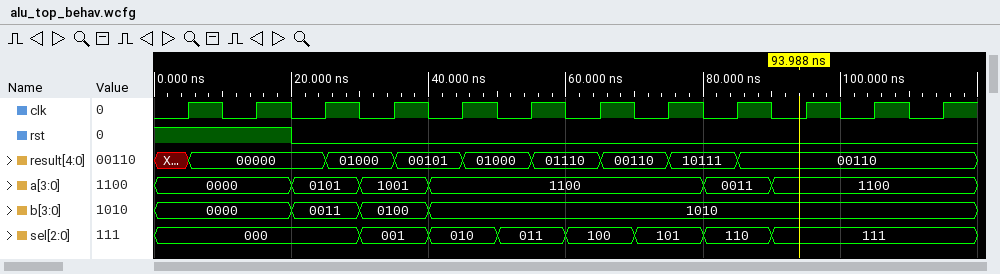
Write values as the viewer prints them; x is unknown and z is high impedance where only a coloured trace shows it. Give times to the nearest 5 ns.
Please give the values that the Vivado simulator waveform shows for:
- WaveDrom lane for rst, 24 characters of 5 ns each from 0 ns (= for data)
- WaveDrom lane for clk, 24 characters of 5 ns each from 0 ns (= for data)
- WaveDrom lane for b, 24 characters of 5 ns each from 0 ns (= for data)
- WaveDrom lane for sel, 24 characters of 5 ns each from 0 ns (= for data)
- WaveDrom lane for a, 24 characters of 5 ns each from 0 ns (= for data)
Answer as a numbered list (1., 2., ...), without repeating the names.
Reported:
1. {name: 'rst', wave: '1...0...................'}
2. {name: 'clk', wave: '010101010101010101010101'}
3. {name: 'b', wave: '=...=.=.=...............', data: '0000 0011 0100 1010'}
4. {name: 'sel', wave: '=.....=.=.=.=.=.=.=.....', data: '000 001 010 011 100 101 110 111'}
5. {name: 'a', wave: '=...=.=.=.......=.=.....', data: '0000 0101 1001 1100 0011 1100'}
